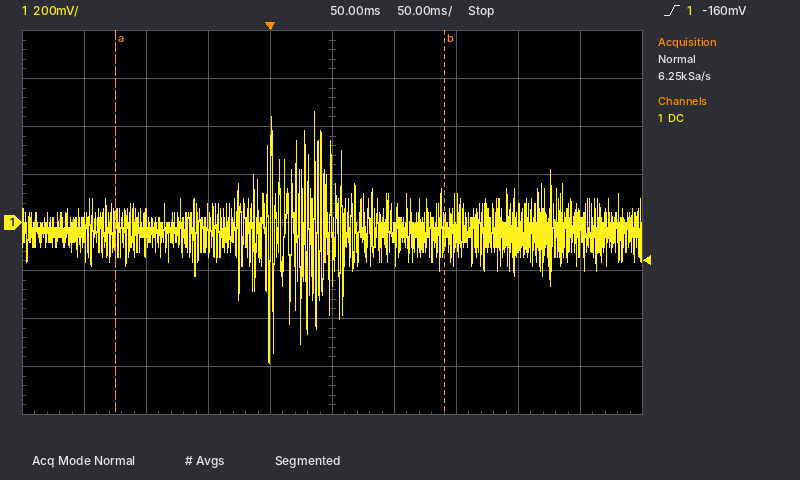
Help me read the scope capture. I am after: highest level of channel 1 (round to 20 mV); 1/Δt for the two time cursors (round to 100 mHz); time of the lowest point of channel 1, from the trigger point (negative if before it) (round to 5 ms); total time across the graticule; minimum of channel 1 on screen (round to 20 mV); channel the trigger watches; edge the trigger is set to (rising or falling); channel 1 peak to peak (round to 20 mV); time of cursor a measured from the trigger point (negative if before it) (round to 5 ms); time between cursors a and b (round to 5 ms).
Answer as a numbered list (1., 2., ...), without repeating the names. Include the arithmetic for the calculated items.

1. 460 mV
2. 1 / 265 ms ≈ 3.8 Hz
3. 0 ms
4. 500 ms
5. -580 mV
6. channel 1
7. rising
8. 460 mV − (-580 mV) = 1.04 V
9. -125 ms
10. 265 ms
